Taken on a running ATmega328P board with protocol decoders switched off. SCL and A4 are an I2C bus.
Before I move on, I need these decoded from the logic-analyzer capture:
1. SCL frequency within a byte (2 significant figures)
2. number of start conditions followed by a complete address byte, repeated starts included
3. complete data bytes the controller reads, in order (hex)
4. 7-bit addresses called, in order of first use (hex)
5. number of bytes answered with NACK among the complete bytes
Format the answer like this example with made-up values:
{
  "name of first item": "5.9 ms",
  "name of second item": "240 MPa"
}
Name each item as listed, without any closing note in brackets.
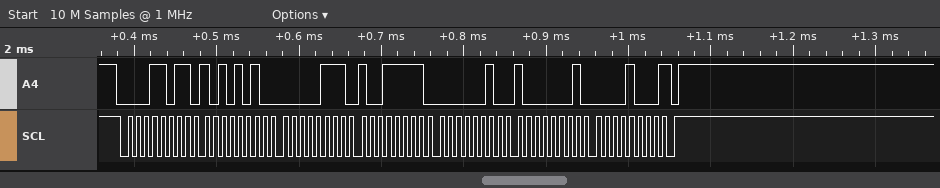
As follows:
{
  "SCL frequency within a byte": "100 kHz",
  "number of start conditions followed by a complete address byte, repeated starts included": "1",
  "complete data bytes the controller reads, in order": "AA 07 9F 02 81 08",
  "7-bit addresses called, in order of first use": "0x0D",
  "number of bytes answered with NACK among the complete bytes": "1"
}
